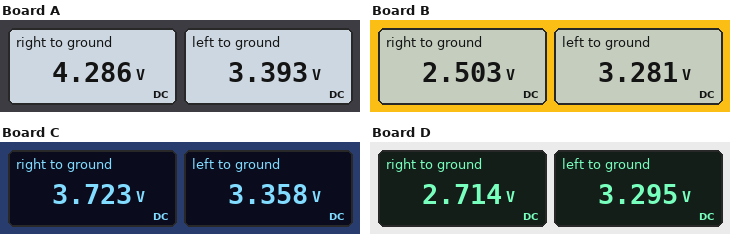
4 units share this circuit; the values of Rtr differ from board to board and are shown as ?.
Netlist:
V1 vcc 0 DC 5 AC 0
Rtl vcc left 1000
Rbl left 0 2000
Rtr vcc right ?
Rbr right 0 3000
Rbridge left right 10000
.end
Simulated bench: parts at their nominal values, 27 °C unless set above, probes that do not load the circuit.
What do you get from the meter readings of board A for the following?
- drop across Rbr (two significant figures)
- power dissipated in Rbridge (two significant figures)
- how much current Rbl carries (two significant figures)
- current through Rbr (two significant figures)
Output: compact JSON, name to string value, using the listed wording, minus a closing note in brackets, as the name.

{"drop across Rbr": "4.3 V", "power dissipated in Rbridge": "80 µW", "how much current Rbl carries": "1.7 mA", "current through Rbr": "1.4 mA"}
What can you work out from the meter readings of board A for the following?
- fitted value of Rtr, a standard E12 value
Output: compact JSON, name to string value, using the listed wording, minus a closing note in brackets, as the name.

{"fitted value of Rtr, a standard E12 value": "470 Ω"}
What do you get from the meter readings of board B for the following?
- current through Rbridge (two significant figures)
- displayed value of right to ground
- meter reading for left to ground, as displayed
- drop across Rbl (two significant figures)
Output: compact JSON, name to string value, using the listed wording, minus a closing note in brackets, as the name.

{"current through Rbridge": "78 µA", "displayed value of right to ground": "2.503 V", "meter reading for left to ground, as displayed": "3.281 V", "drop across Rbl": "3.3 V"}
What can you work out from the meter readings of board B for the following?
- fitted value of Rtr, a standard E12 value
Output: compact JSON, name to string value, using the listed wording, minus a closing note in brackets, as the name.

{"fitted value of Rtr, a standard E12 value": "3.3 kΩ"}
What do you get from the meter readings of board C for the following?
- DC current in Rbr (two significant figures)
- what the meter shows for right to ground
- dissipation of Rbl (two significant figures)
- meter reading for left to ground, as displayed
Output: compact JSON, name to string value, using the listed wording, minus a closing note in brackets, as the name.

{"DC current in Rbr": "1.2 mA", "what the meter shows for right to ground": "3.723 V", "dissipation of Rbl": "5.6 mW", "meter reading for left to ground, as displayed": "3.358 V"}
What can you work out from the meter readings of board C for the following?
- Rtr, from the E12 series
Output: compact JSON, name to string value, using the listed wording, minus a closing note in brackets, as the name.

{"Rtr, from the E12 series": "1 kΩ"}
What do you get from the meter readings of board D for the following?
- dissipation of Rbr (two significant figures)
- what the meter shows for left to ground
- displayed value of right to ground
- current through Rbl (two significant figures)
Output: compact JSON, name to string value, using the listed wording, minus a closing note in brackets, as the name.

{"dissipation of Rbr": "2.5 mW", "what the meter shows for left to ground": "3.295 V", "displayed value of right to ground": "2.714 V", "current through Rbl": "1.6 mA"}
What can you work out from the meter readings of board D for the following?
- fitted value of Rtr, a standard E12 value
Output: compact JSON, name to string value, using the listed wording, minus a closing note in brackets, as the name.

{"fitted value of Rtr, a standard E12 value": "2.7 kΩ"}
